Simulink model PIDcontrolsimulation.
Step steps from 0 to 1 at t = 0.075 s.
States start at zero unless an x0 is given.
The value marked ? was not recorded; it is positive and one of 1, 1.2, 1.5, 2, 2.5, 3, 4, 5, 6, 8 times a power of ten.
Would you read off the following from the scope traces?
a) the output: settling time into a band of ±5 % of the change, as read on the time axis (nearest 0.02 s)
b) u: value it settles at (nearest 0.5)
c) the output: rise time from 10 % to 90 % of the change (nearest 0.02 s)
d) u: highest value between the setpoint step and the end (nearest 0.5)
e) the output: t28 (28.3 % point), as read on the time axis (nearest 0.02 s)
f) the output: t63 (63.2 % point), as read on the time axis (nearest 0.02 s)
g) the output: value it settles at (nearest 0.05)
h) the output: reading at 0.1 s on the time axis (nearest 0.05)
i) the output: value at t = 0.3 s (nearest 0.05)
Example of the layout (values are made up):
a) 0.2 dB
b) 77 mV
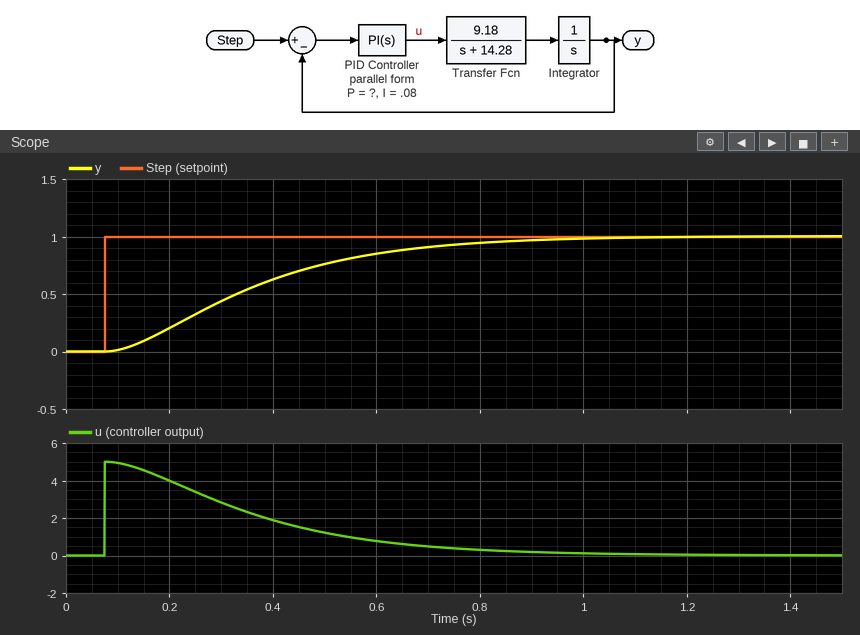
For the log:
a) 0.84 s
b) 0.0
c) 0.54 s
d) 5.0
e) 0.24 s
f) 0.40 s
g) 1.00
h) 0.00
i) 0.45
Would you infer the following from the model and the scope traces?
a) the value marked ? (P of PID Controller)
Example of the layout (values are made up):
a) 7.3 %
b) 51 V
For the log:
a) 5
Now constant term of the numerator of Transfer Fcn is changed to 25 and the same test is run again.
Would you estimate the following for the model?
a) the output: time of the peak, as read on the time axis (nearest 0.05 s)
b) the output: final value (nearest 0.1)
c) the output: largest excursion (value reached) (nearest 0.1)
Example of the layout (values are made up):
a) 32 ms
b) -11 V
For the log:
a) 0.45 s
b) 1.0
c) 1.1
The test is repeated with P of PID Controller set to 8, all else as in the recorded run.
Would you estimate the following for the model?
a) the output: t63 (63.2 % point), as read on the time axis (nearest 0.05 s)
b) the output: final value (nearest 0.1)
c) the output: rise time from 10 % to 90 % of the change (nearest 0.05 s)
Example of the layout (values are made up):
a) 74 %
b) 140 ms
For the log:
a) 0.30 s
b) 1.0
c) 0.30 s
